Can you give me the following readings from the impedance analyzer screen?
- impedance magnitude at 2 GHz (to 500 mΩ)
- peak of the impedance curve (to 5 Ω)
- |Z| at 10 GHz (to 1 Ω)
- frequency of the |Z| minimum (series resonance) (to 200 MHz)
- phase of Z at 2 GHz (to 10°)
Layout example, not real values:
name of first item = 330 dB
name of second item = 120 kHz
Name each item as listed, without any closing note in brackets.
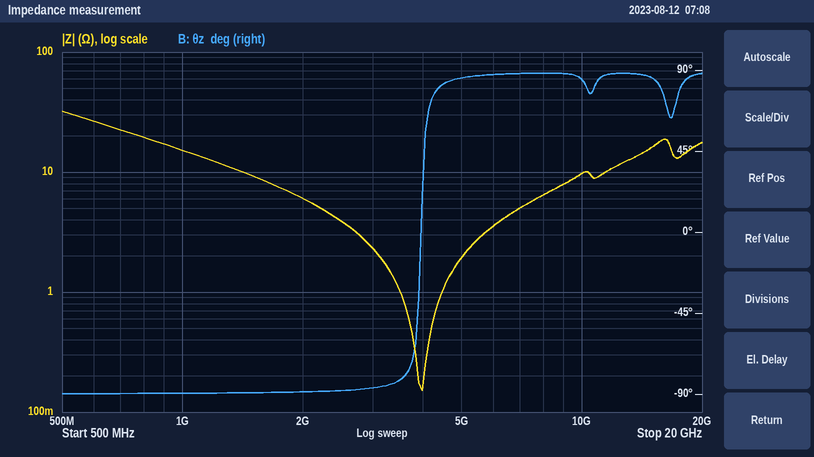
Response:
impedance magnitude at 2 GHz = 6.0 Ω
peak of the impedance curve = 30 Ω
|Z| at 10 GHz = 10 Ω
frequency of the |Z| minimum (series resonance) = 4.0 GHz
phase of Z at 2 GHz = -90°
